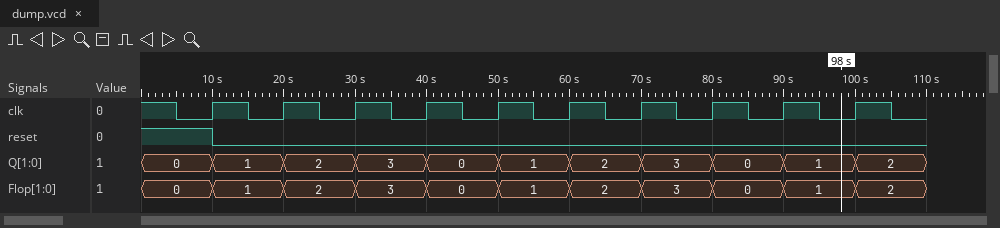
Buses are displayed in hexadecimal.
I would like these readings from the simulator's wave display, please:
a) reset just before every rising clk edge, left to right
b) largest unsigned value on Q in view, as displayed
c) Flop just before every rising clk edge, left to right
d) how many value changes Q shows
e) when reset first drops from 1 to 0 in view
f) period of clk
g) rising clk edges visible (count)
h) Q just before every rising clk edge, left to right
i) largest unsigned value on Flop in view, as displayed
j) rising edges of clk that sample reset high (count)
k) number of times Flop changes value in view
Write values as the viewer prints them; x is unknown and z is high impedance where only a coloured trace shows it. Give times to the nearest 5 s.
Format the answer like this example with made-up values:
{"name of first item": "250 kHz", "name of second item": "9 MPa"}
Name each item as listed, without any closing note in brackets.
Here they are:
{"reset just before every rising clk edge, left to right": "1 0 0 0 0 0 0 0 0 0", "largest unsigned value on Q in view, as displayed": "3", "Flop just before every rising clk edge, left to right": "0, 1, 2, 3, 0, 1, 2, 3, 0, 1", "how many value changes Q shows": "10", "when reset first drops from 1 to 0 in view": "10 s", "period of clk": "10 s", "rising clk edges visible": "10", "Q just before every rising clk edge, left to right": "0, 1, 2, 3, 0, 1, 2, 3, 0, 1", "largest unsigned value on Flop in view, as displayed": "3", "rising edges of clk that sample reset high": "1", "number of times Flop changes value in view": "10"}
